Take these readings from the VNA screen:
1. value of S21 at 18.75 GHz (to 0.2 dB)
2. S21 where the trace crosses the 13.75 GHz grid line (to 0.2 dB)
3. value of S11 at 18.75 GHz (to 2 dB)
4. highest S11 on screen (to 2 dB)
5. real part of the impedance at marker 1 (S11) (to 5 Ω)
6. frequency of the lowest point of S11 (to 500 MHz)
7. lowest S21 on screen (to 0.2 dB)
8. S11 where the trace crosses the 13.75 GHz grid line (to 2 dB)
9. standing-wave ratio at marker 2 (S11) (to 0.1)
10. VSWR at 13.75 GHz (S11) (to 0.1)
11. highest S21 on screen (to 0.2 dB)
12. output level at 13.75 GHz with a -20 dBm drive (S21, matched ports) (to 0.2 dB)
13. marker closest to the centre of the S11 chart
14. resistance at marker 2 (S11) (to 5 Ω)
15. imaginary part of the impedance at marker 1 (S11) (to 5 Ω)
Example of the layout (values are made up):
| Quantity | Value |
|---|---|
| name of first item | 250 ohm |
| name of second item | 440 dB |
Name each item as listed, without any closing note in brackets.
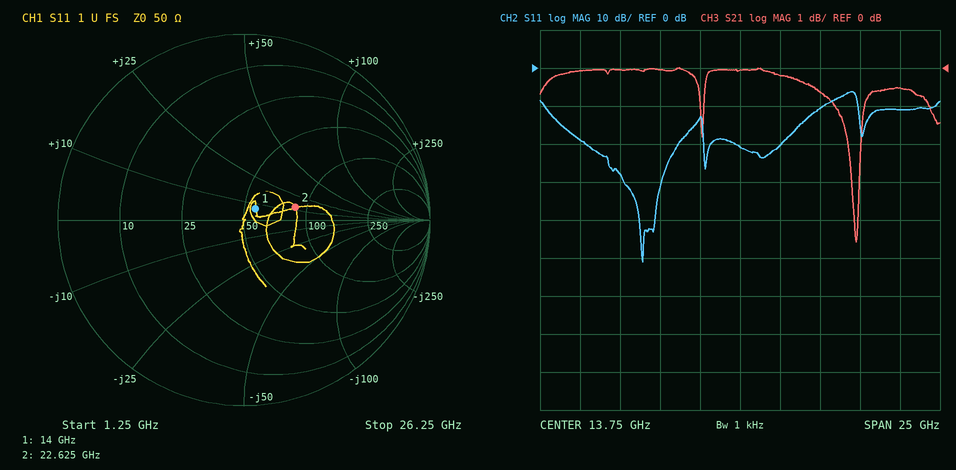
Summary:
| Quantity | Value |
|---|---|
| value of S21 at 18.75 GHz | -0.6 dB |
| S21 where the trace crosses the 13.75 GHz grid line | 0.0 dB |
| value of S11 at 18.75 GHz | -10 dB |
| highest S11 on screen | -6 dB |
| real part of the impedance at marker 1 (S11) | 55 Ω |
| frequency of the lowest point of S11 | 7.5 GHz |
| lowest S21 on screen | -4.6 dB |
| S11 where the trace crosses the 13.75 GHz grid line | -20 dB |
| standing-wave ratio at marker 2 (S11) | 1.8 |
| VSWR at 13.75 GHz (S11) | 1.2 |
| highest S21 on screen | 0.0 dB |
| output level at 13.75 GHz with a -20 dBm drive (S21, matched ports) | -20.0 dBm |
| marker closest to the centre of the S11 chart | marker 1 |
| resistance at marker 2 (S11) | 85 Ω |
| imaginary part of the impedance at marker 1 (S11) | +5 Ω |
